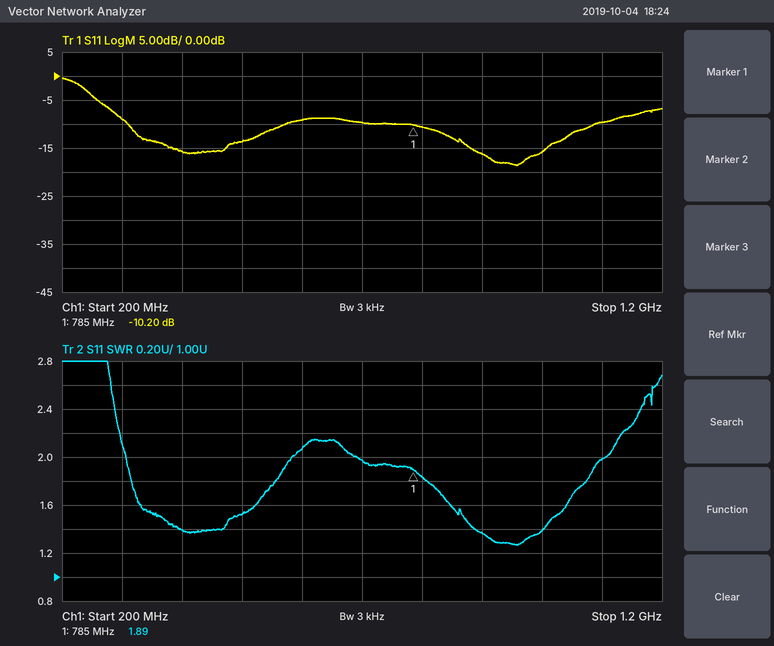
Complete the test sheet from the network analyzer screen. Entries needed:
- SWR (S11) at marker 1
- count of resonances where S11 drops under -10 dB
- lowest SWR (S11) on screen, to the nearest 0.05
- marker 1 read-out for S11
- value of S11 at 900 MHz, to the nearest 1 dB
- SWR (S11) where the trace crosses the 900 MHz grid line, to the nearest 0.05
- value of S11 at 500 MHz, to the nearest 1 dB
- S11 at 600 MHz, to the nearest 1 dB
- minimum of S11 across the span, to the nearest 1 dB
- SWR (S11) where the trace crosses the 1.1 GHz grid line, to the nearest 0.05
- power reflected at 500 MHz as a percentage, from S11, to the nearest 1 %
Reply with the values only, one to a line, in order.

1.89
2
1.25
-10.20 dB
-16 dB
1.35
-14 dB
-9 dB
-19 dB
2.00
4 %
